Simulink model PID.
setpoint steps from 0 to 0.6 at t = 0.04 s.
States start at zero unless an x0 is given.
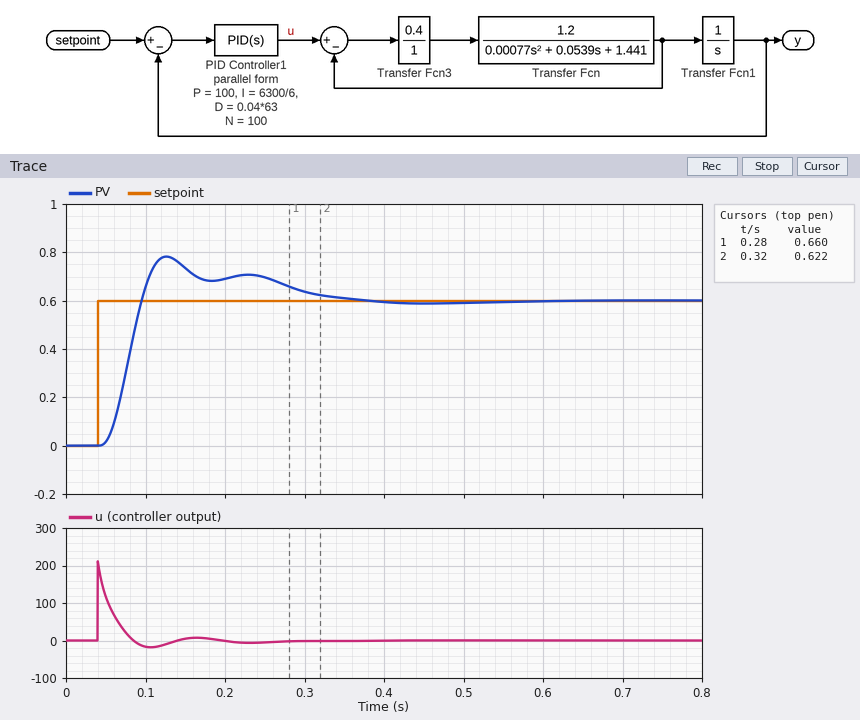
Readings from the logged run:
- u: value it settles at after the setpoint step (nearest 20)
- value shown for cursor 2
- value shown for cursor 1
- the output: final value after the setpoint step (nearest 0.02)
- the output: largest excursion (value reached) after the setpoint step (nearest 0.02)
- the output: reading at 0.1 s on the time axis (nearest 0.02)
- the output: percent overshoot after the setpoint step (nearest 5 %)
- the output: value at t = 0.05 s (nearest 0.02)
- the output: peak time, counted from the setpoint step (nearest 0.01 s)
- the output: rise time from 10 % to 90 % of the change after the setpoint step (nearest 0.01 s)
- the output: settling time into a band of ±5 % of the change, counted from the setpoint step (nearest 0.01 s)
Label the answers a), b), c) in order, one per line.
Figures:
a) 0
b) 0.622
c) 0.660
d) 0.60
e) 0.78
f) 0.66
g) 30 %
h) 0.02
i) 0.09 s
j) 0.03 s
k) 0.27 s
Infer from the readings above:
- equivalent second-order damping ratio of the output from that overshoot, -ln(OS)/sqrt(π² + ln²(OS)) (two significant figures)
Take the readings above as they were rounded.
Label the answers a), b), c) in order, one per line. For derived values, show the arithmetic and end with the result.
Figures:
a) ln(0.3) = -1.204; 1.204 / sqrt(9.870 + 1.450) = 0.36
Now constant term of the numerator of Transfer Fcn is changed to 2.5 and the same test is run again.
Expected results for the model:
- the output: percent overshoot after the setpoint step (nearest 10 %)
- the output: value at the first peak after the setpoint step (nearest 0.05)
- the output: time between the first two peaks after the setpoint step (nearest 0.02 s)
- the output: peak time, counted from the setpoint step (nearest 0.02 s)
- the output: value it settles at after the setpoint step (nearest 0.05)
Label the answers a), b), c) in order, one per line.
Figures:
a) 50 %
b) 0.90
c) 0.10 s
d) 0.06 s
e) 0.60
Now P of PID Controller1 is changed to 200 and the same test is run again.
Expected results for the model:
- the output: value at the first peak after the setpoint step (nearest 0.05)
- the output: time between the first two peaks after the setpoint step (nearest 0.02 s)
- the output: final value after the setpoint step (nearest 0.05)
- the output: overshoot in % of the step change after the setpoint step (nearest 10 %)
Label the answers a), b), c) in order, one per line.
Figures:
a) 0.95
b) 0.12 s
c) 0.60
d) 60 %
